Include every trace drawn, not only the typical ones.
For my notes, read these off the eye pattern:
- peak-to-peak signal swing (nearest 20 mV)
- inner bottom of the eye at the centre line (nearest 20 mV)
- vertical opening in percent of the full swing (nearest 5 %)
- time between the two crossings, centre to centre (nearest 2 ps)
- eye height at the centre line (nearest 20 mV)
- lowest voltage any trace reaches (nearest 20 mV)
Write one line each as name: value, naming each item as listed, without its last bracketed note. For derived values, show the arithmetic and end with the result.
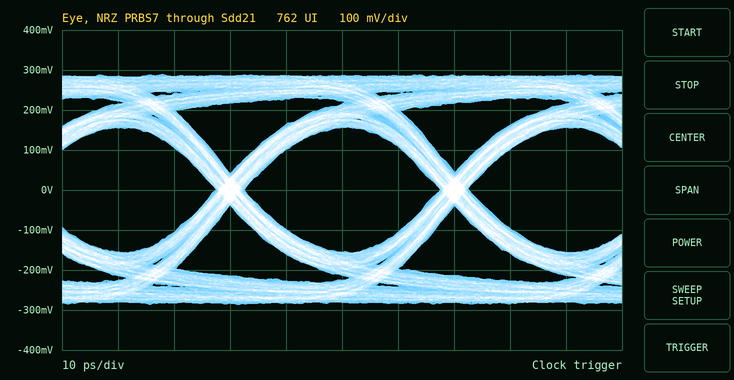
peak-to-peak signal swing: 580 mV
inner bottom of the eye at the centre line: -160 mV
vertical opening in percent of the full swing: 320 mV / 580 mV ≈ 55 %
time between the two crossings, centre to centre: 40 ps
eye height at the centre line: 320 mV
lowest voltage any trace reaches: -280 mV
